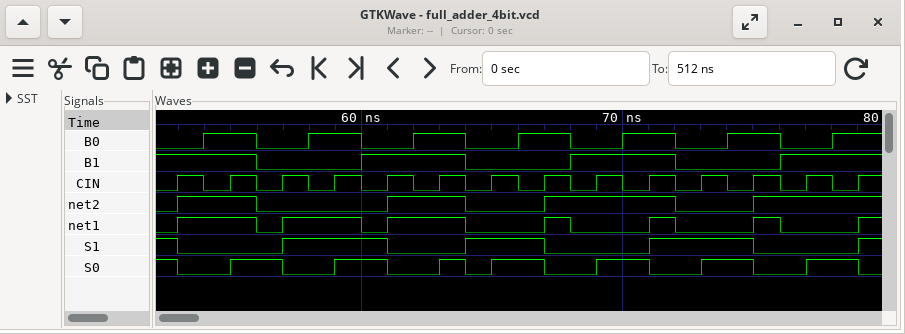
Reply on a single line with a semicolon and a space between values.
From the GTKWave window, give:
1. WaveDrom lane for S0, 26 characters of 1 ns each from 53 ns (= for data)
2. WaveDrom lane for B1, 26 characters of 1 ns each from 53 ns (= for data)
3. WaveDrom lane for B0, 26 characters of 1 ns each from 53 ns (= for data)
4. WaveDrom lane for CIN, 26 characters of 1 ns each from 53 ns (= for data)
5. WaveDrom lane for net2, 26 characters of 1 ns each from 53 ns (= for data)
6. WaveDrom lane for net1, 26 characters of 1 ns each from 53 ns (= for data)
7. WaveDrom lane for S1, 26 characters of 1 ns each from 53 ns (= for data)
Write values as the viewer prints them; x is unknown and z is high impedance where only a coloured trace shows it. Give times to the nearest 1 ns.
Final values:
{name: 'S0', wave: '0.1.0.1.0.101.0.1.0.1.0.1.'}; {name: 'B1', wave: '1..0...1...0...1...0...1..'}; {name: 'B0', wave: '01.0.1.0.1.0.1.0.1.0.1.0.1'}; {name: 'CIN', wave: '10101010101010101010101010'}; {name: 'net2', wave: '1..0....1..0..1....0..1...'}; {name: 'net1', wave: '1..01..01..0..10..10..10..'}; {name: 'S1', wave: '0...1...0..1..0...1...0...'}
